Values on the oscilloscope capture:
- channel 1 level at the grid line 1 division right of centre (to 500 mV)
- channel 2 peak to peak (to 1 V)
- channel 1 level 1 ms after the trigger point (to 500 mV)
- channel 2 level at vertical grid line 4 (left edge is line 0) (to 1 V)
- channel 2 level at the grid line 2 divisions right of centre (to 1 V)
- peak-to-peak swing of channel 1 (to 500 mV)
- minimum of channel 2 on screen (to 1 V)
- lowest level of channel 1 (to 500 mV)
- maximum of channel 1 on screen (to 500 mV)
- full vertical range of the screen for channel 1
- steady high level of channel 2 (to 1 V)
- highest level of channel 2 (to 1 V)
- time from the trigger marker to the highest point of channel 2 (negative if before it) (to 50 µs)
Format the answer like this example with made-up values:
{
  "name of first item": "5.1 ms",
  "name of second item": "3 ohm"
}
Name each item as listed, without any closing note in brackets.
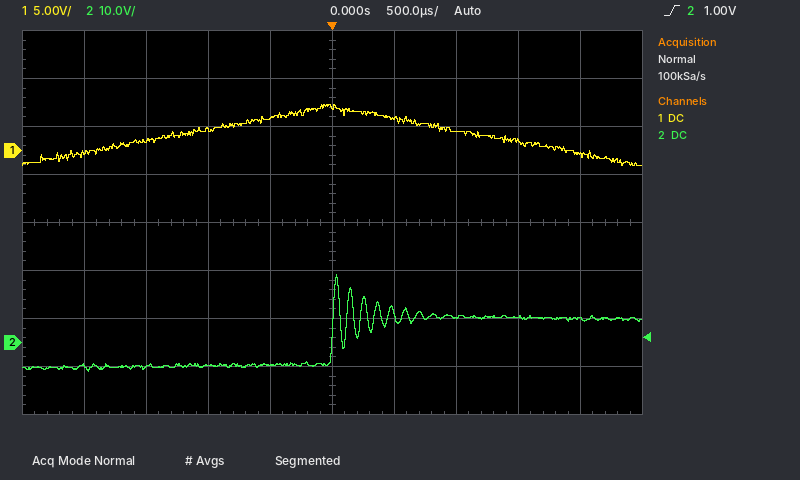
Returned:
{
  "channel 1 level at the grid line 1 division right of centre": "3.5 V",
  "channel 2 peak to peak": "20 V",
  "channel 1 level 1 ms after the trigger point": "2.0 V",
  "channel 2 level at vertical grid line 4 (left edge is line 0)": "-5 V",
  "channel 2 level at the grid line 2 divisions right of centre": "5 V",
  "peak-to-peak swing of channel 1": "6.5 V",
  "minimum of channel 2 on screen": "-6 V",
  "lowest level of channel 1": "-1.5 V",
  "maximum of channel 1 on screen": "5.0 V",
  "full vertical range of the screen for channel 1": "40 V",
  "steady high level of channel 2": "5 V",
  "highest level of channel 2": "14 V",
  "time from the trigger marker to the highest point of channel 2 (negative if before it)": "+50 µs"
}
